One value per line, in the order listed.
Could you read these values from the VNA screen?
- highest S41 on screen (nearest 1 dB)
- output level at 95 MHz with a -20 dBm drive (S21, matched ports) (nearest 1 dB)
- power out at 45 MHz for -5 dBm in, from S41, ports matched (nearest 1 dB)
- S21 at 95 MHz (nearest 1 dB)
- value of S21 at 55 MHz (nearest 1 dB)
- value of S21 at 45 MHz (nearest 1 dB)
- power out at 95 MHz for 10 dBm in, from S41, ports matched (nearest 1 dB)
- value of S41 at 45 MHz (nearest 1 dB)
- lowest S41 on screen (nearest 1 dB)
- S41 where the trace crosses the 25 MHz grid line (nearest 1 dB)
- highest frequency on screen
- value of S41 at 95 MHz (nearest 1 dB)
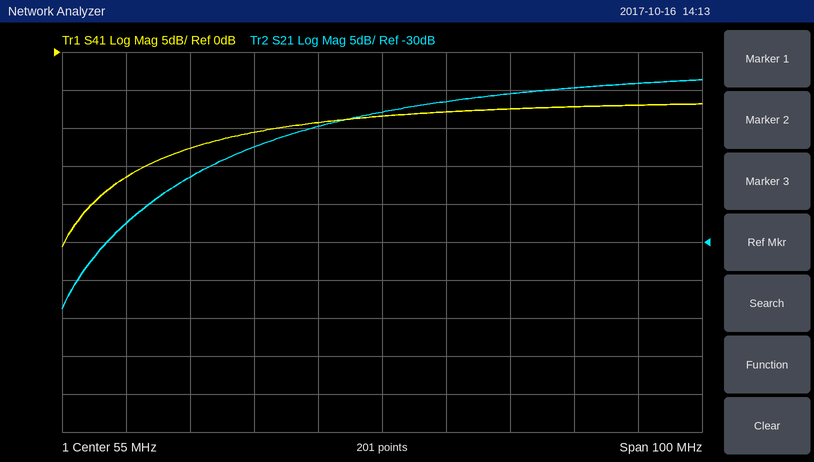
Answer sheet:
-7 dB
-29 dBm
-14 dBm
-9 dB
-13 dB
-15 dB
3 dBm
-9 dB
-26 dB
-13 dB
105 MHz
-7 dB
